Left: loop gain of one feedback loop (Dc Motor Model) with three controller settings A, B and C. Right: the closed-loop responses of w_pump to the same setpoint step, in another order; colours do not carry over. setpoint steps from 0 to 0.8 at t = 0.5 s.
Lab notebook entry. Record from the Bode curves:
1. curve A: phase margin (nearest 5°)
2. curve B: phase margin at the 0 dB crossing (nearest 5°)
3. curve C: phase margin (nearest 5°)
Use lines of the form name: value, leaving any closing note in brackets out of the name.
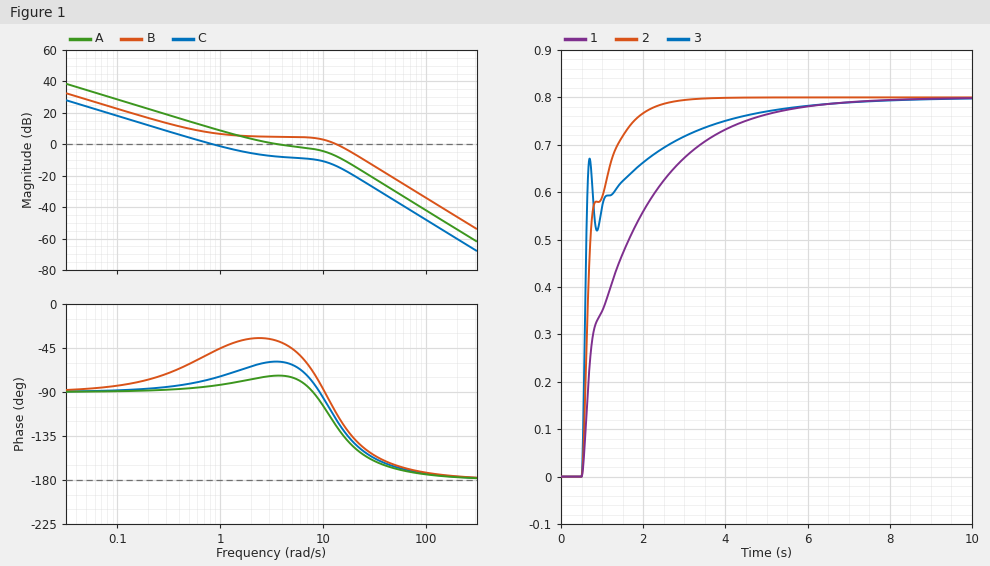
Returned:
curve A: phase margin: 105°
curve B: phase margin at the 0 dB crossing: 70°
curve C: phase margin: 105°
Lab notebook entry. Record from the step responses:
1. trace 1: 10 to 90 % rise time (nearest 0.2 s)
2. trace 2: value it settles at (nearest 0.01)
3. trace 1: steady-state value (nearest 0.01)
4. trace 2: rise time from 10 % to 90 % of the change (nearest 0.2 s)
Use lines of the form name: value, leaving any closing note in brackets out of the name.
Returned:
trace 1: 10 to 90 % rise time: 3.2 s
trace 2: value it settles at: 0.80
trace 1: steady-state value: 0.80
trace 2: rise time from 10 % to 90 % of the change: 1.0 s
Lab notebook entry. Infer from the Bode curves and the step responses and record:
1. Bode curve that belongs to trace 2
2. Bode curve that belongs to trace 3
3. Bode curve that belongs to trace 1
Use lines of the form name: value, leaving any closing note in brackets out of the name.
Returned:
Bode curve that belongs to trace 2: A
Bode curve that belongs to trace 3: B
Bode curve that belongs to trace 1: C
